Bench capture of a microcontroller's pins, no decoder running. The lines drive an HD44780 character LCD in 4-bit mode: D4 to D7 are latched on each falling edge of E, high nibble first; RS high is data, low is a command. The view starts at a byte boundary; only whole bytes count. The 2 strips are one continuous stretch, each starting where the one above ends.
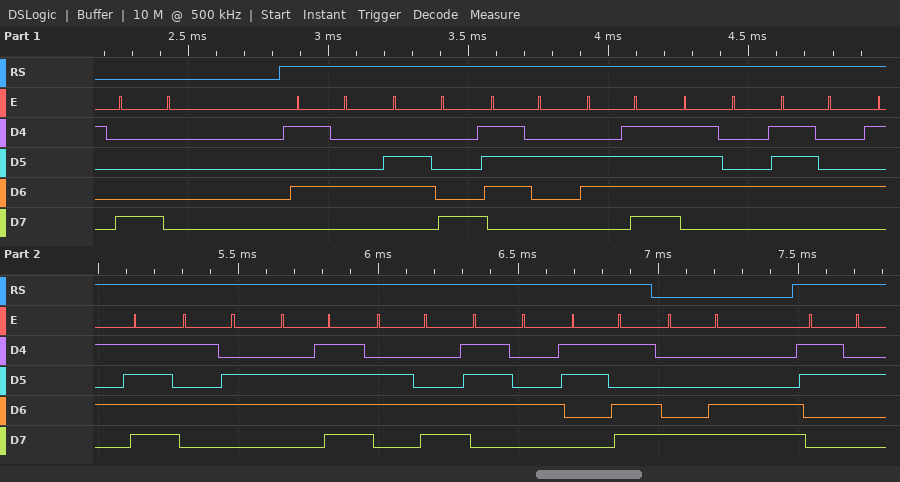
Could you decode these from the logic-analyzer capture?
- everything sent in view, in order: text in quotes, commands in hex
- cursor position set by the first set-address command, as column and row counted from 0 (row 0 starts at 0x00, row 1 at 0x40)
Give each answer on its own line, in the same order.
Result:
0x80 "Thrott_Volt=" 0x8C "2"
column 0, row 0
